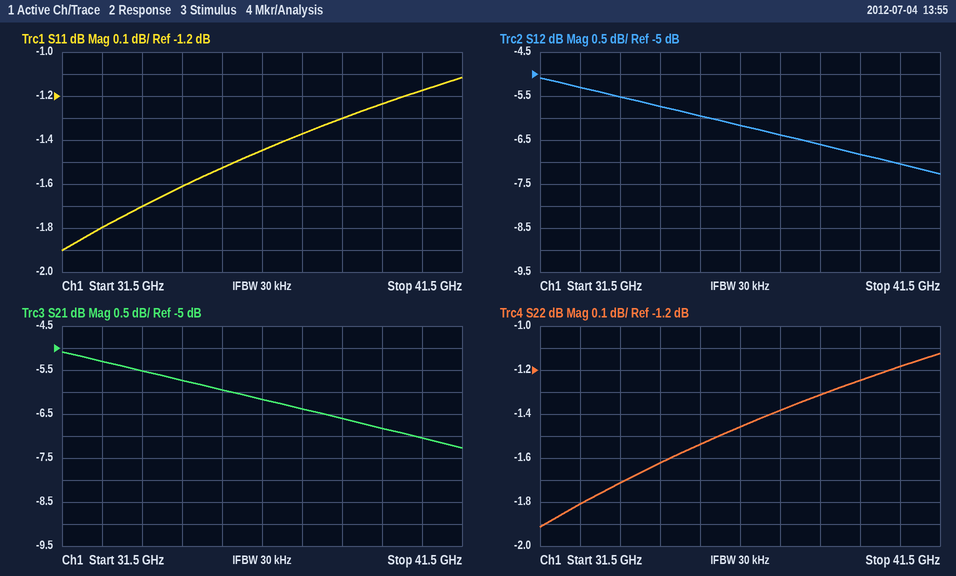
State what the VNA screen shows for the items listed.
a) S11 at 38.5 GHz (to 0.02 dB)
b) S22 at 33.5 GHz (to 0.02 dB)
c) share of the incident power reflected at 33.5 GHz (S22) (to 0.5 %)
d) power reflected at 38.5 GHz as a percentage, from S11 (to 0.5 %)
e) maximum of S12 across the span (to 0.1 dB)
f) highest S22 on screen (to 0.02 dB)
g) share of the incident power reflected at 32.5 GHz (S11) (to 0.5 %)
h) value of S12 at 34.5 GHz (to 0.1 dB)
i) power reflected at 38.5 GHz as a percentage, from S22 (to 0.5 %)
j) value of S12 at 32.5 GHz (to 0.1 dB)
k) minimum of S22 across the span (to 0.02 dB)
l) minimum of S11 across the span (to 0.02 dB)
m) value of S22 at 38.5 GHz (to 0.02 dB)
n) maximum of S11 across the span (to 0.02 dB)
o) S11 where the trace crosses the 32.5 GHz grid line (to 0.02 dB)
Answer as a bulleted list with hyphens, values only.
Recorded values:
- -1.30 dB
- -1.72 dB
- 67.5 %
- 74.0 %
- -5.1 dB
- -1.12 dB
- 66.0 %
- -5.7 dB
- 74.0 %
- -5.3 dB
- -1.92 dB
- -1.90 dB
- -1.32 dB
- -1.12 dB
- -1.80 dB
